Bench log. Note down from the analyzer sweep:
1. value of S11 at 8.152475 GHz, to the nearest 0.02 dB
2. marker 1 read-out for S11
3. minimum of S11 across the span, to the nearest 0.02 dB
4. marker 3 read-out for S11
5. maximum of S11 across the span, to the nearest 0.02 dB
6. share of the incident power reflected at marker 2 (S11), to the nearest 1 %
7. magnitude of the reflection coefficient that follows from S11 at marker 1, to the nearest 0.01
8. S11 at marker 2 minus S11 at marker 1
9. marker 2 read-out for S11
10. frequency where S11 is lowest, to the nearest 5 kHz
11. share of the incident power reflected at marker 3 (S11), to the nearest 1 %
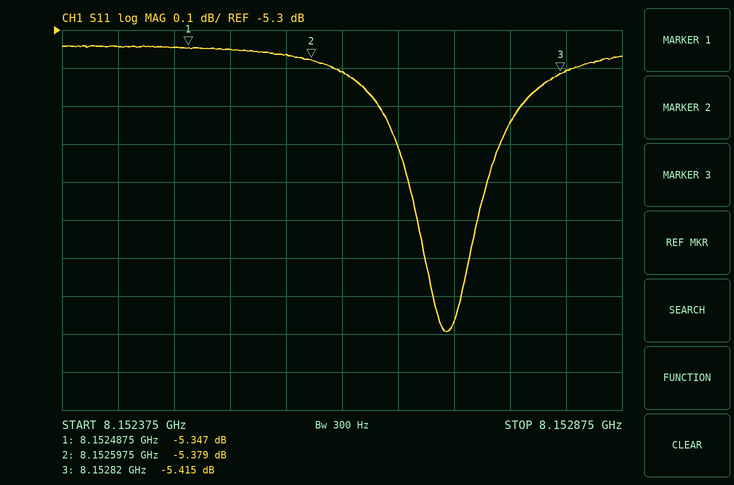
-5.34 dB
-5.347 dB
-6.10 dB
-5.415 dB
-5.34 dB
29 %
0.54
-0.032 dB
-5.379 dB
8.152720 GHz
29 %
